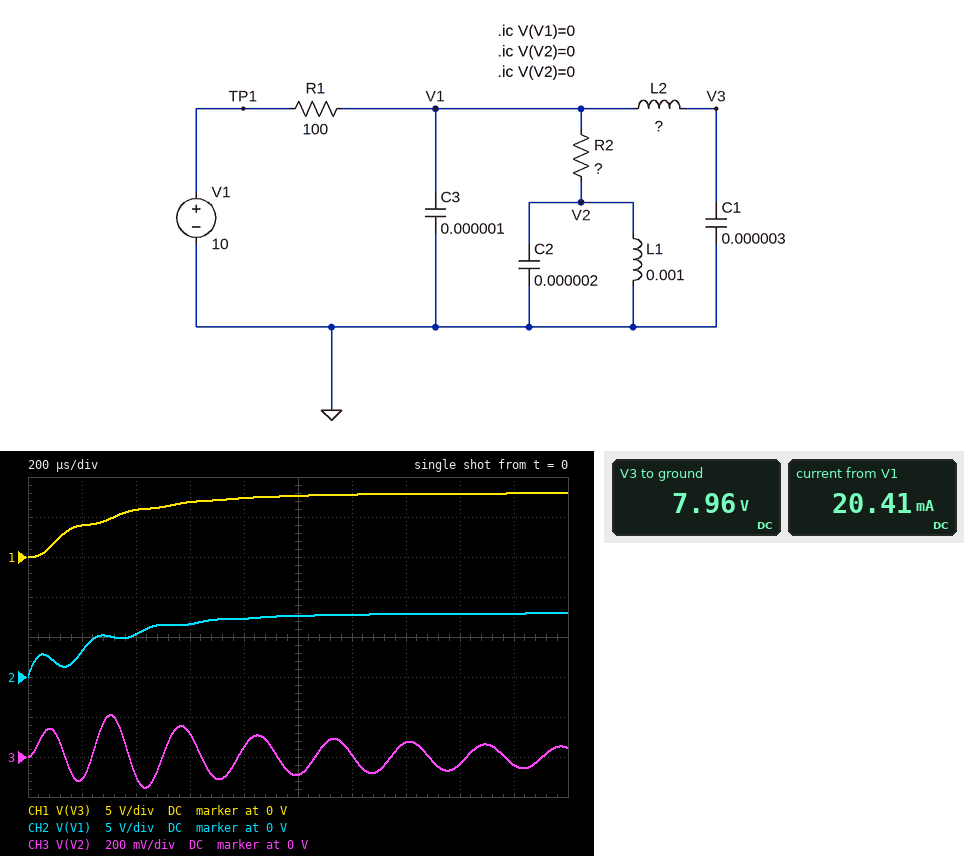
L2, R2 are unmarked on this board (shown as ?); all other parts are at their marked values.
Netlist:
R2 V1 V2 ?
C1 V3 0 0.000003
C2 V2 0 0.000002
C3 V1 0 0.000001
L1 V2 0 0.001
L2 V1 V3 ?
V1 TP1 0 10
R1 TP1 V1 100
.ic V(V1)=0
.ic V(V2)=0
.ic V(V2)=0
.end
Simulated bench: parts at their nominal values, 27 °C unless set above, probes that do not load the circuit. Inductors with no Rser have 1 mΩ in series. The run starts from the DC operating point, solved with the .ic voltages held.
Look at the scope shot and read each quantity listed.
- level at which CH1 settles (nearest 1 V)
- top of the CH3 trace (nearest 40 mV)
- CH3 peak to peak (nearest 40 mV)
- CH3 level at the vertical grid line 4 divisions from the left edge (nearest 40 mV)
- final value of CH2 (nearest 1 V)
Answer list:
8 V
200 mV
360 mV
40 mV
8 V
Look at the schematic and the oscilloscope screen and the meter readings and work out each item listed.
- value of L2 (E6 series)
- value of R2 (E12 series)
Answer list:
1.5 mH
390 Ω
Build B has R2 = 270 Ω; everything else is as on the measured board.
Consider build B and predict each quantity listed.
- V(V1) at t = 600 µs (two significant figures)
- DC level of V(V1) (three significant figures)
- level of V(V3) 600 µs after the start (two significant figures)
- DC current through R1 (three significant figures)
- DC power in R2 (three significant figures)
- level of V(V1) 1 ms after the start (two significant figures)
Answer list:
6.2 V
7.30 V
6.5 V
27.0 mA
197 mW
7.1 V
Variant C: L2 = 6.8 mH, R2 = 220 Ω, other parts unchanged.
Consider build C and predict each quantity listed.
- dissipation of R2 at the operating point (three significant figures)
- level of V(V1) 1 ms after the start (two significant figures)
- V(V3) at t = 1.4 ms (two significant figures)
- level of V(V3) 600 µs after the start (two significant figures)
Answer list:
215 mW
6.8 V
6.9 V
6.4 V
